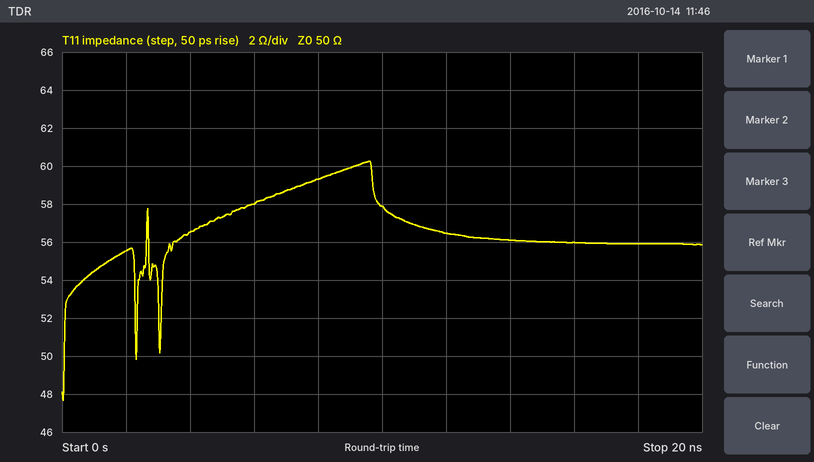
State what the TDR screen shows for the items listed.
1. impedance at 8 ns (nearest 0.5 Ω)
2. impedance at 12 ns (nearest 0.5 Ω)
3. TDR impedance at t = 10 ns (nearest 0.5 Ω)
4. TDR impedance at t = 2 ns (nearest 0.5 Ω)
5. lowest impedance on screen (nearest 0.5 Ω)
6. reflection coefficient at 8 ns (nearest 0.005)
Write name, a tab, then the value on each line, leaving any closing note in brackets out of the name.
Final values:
impedance at 8 ns	59.5 Ω
impedance at 12 ns	56.5 Ω
TDR impedance at t = 10 ns	58.0 Ω
TDR impedance at t = 2 ns	55.5 Ω
lowest impedance on screen	47.5 Ω
reflection coefficient at 8 ns	+0.085
